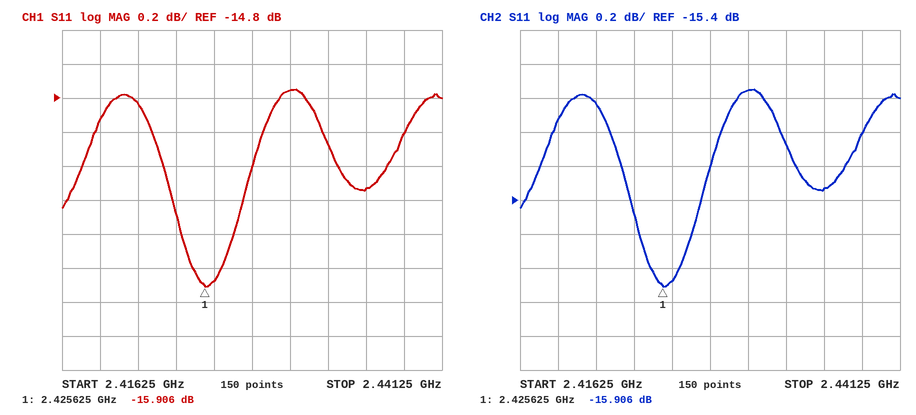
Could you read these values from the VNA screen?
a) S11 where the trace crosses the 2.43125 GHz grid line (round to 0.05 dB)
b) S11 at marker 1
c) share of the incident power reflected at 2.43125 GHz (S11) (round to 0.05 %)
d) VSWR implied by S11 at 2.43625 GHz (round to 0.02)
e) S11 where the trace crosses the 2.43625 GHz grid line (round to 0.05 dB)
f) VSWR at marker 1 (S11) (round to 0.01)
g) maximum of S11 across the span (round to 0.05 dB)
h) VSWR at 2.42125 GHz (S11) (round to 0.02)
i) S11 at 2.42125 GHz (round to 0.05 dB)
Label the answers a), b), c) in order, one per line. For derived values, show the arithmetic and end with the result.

a) -14.75 dB
b) -15.906 dB
c) 10^(-14.75/10) ≈ 3.35 %
d) |Γ| = 10^(-15.35/20) = 0.1708; VSWR = (1 + 0.1708)/(1 − 0.1708) ≈ 1.41, so 1.42 to the nearest 0.02
e) -15.35 dB
f) (1 + 0.1602)/(1 − 0.1602) ≈ 1.38
g) -14.75 dB
h) |Γ| = 10^(-14.85/20) = 0.1809; VSWR = (1 + 0.1809)/(1 − 0.1809) ≈ 1.44
i) -14.85 dB
